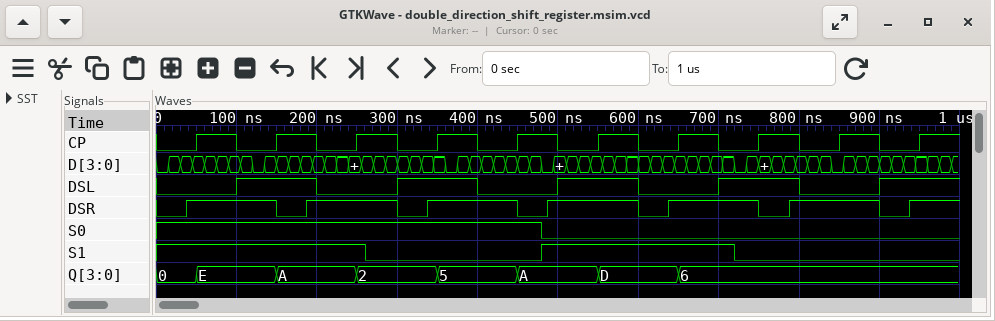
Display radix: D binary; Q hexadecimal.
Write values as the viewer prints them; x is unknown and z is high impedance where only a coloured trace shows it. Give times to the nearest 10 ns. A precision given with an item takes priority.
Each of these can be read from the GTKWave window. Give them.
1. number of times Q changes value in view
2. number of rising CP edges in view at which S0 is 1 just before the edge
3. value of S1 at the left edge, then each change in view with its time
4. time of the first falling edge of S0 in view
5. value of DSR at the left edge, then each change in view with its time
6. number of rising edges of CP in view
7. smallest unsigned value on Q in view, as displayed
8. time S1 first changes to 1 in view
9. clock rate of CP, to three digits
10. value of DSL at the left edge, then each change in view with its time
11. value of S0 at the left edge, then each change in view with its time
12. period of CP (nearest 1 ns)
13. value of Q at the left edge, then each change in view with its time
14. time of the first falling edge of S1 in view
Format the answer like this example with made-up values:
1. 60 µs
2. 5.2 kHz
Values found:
1. 7
2. 5
3. 1, 0 at 260 ns, 1 at 480 ns, 0 at 720 ns
4. 480 ns
5. 0, 1 at 40 ns, 0 at 150 ns, 1 at 190 ns, 0 at 300 ns, 1 at 340 ns, 0 at 450 ns, 1 at 490 ns, 0 at 600 ns, 1 at 640 ns, 0 at 750 ns, 1 at 790 ns, 0 at 900 ns, 1 at 940 ns
6. 10
7. 0
8. 480 ns
9. 10.0 MHz
10. 0, 1 at 100 ns, 0 at 200 ns, 1 at 300 ns, 0 at 400 ns, 1 at 500 ns, 0 at 600 ns, 1 at 700 ns, 0 at 800 ns, 1 at 900 ns
11. 1, 0 at 480 ns
12. 100 ns
13. 0, E at 50 ns, A at 150 ns, 2 at 250 ns, 5 at 350 ns, A at 450 ns, D at 550 ns, 6 at 650 ns
14. 260 ns
